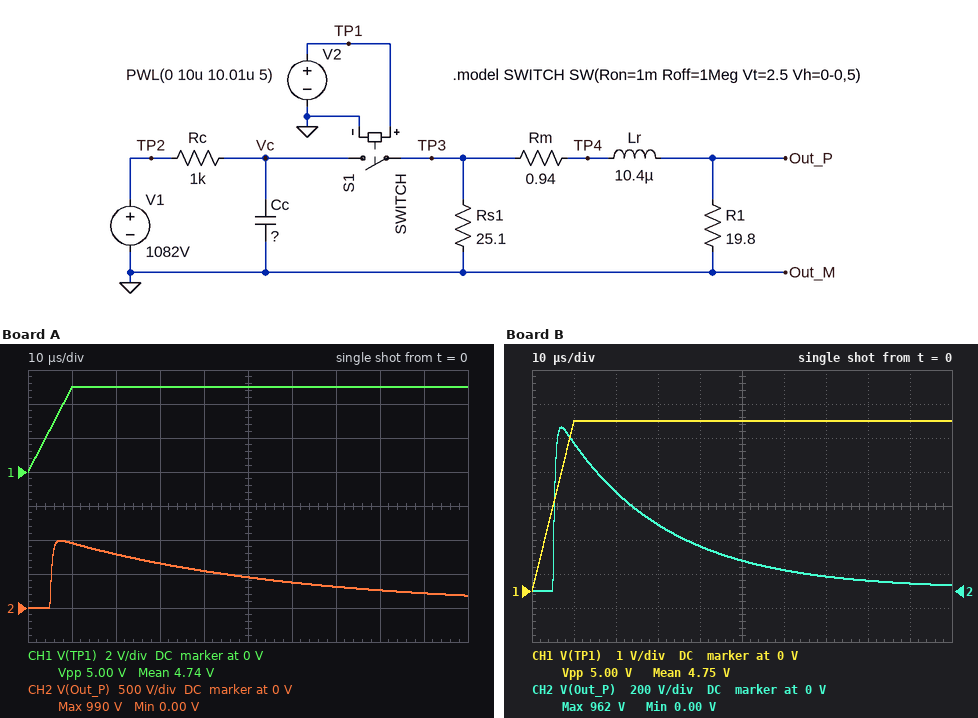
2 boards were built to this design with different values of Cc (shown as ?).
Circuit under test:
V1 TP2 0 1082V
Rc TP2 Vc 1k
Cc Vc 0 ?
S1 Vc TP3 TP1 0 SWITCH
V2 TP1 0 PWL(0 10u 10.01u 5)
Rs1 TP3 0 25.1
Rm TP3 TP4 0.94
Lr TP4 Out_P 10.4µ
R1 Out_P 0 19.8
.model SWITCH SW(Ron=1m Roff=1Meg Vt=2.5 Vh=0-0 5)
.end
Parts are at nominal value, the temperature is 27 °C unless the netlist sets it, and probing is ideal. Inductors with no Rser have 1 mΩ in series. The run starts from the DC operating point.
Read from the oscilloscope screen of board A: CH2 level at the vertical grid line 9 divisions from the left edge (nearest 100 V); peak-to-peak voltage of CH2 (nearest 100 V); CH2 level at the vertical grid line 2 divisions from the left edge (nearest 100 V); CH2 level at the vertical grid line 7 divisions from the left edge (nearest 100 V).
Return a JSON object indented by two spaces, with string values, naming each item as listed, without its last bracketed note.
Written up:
{
  "CH2 level at the vertical grid line 9 divisions from the left edge": "200 V",
  "peak-to-peak voltage of CH2": "1.0 kV",
  "CH2 level at the vertical grid line 2 divisions from the left edge": "800 V",
  "CH2 level at the vertical grid line 7 divisions from the left edge": "300 V"
}
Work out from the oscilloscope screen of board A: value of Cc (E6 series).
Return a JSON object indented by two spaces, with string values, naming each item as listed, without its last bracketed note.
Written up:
{
  "value of Cc": "4.7 µF"
}
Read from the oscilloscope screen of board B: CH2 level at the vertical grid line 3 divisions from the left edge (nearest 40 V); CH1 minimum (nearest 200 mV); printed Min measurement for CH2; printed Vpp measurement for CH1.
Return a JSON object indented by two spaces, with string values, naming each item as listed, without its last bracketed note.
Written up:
{
  "CH2 level at the vertical grid line 3 divisions from the left edge": "400 V",
  "CH1 minimum": "0 V",
  "printed Min measurement for CH2": "0.00 V",
  "printed Vpp measurement for CH1": "5.00 V"
}
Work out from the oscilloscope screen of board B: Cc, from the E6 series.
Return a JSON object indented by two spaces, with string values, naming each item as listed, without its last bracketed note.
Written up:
{
  "Cc, from the E6 series": "2.2 µF"
}
